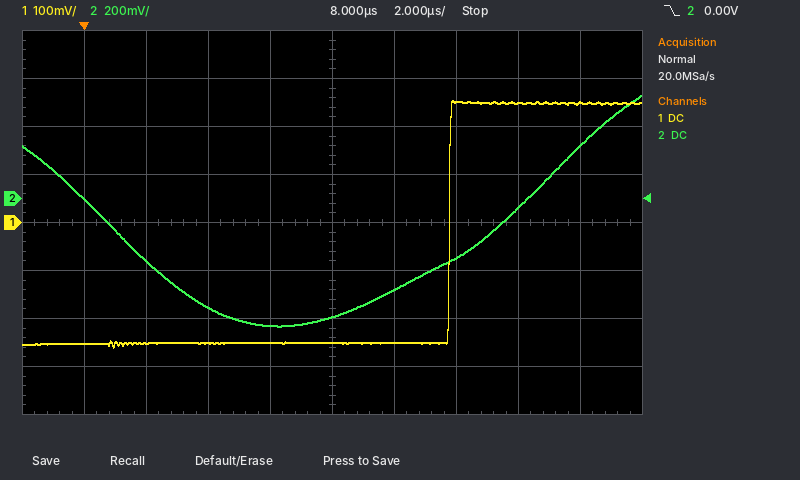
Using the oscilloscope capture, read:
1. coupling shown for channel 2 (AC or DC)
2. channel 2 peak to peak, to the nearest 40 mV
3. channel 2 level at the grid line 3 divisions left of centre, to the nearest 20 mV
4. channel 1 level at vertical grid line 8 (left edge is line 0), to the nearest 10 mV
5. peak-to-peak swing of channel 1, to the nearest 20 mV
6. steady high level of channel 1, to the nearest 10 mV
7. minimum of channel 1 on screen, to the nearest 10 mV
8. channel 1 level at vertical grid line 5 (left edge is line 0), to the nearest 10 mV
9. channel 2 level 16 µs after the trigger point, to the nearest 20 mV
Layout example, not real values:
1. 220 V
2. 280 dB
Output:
1. DC
2. 960 mV
3. -260 mV
4. 250 mV
5. 520 mV
6. 250 mV
7. -260 mV
8. -250 mV
9. 220 mV
